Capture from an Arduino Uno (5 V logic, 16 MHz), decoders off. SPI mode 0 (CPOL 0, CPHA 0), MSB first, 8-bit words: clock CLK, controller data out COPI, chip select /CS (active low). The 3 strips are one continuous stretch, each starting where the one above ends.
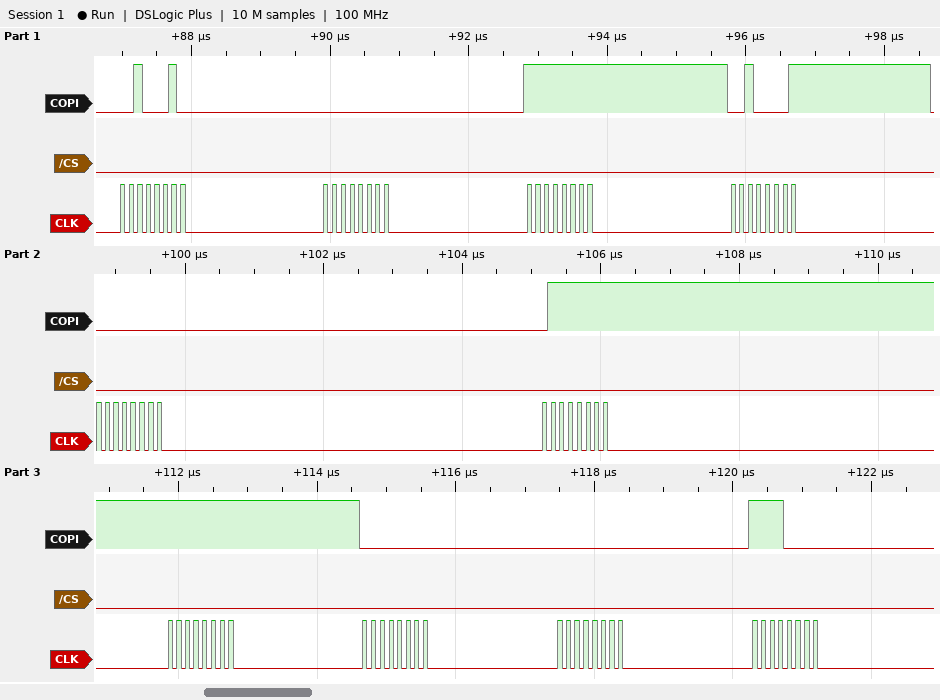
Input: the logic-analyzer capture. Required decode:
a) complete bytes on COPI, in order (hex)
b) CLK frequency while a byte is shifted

22 00 FF 21 00 7F FF 00 00 F0
8 MHz
